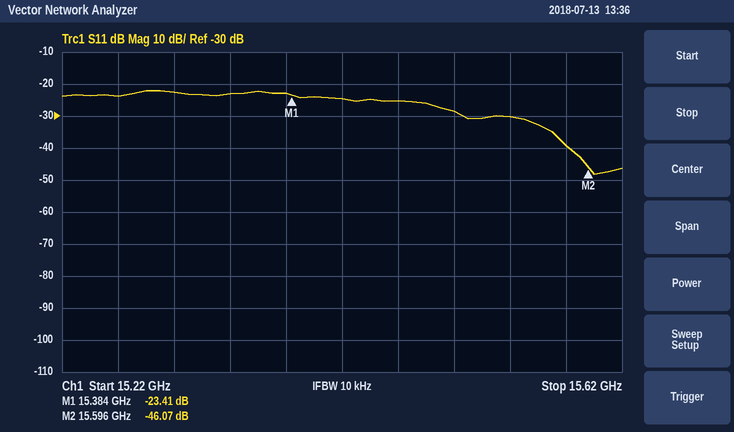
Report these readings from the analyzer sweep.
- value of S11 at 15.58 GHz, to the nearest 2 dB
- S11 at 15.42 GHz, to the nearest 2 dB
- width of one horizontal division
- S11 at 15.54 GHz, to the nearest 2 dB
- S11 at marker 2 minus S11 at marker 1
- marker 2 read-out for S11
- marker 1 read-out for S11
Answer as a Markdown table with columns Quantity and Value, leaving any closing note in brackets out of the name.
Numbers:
| Quantity | Value |
|---|---|
| value of S11 at 15.58 GHz, to the nearest 2 dB | -40 dB |
| S11 at 15.42 GHz, to the nearest 2 dB | -24 dB |
| width of one horizontal division | 40 MHz |
| S11 at 15.54 GHz, to the nearest 2 dB | -30 dB |
| S11 at marker 2 minus S11 at marker 1 | -22.66 dB |
| marker 2 read-out for S11 | -46.07 dB |
| marker 1 read-out for S11 | -23.41 dB |
